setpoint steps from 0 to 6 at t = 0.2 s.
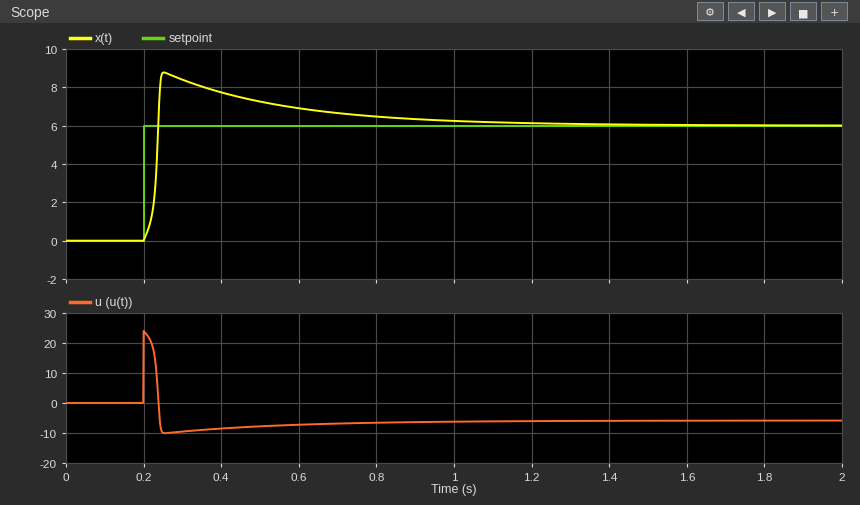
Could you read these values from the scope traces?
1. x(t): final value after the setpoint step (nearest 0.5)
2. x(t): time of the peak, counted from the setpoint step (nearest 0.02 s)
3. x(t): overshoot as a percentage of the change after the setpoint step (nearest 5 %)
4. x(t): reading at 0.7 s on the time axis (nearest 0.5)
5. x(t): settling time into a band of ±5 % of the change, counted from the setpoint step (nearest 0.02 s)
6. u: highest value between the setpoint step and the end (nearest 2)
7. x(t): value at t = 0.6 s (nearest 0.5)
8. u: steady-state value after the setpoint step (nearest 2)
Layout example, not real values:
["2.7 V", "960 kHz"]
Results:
["6.0", "0.06 s", "45 %", "6.5", "0.74 s", "24", "7.0", "-6"]
